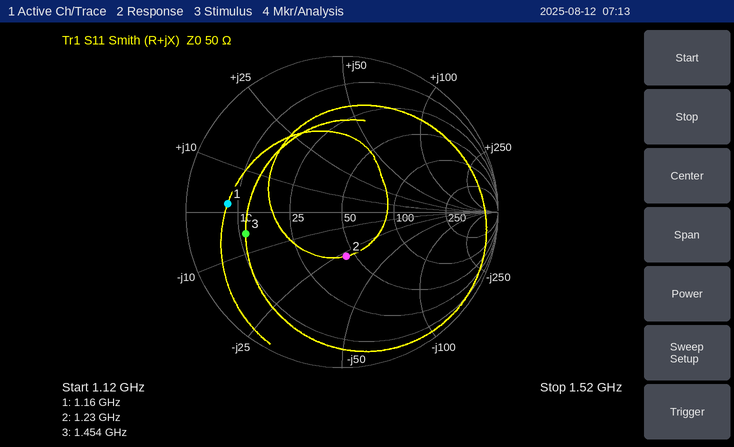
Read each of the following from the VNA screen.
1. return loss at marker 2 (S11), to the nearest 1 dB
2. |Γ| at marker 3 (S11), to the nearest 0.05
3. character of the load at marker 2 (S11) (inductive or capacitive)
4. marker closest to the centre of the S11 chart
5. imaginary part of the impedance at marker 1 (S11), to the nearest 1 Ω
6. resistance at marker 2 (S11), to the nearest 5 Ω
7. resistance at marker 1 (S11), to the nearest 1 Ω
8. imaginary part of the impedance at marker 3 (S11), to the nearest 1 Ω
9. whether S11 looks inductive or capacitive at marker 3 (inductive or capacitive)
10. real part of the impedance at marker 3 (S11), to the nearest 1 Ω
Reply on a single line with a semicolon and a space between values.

11 dB; 0.65; capacitive; marker 2; +2 Ω; 45 Ω; 8 Ω; -5 Ω; capacitive; 11 Ω
